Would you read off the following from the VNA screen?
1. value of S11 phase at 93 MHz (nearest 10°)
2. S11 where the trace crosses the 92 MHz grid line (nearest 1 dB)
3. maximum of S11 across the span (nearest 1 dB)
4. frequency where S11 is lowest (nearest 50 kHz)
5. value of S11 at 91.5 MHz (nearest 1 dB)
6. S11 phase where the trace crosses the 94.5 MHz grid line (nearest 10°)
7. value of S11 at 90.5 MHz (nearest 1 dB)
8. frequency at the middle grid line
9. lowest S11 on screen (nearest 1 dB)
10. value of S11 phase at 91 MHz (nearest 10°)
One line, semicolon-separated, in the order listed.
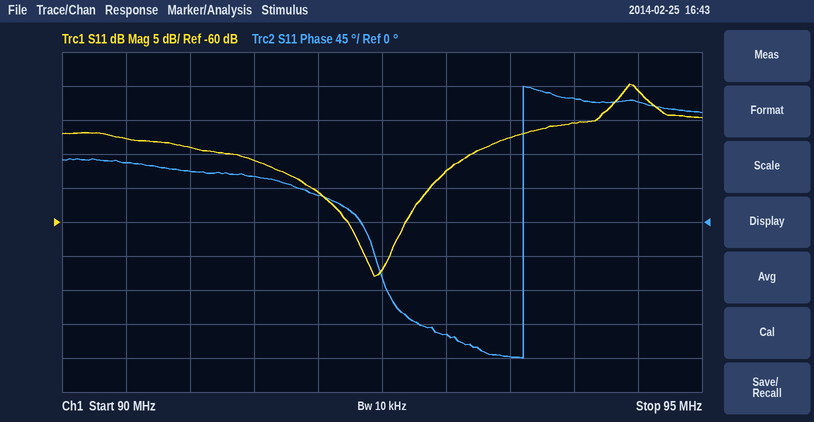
-150°; -56 dB; -40 dB; 92.45 MHz; -51 dB; 160°; -48 dB; 92.5 MHz; -68 dB; 70°
